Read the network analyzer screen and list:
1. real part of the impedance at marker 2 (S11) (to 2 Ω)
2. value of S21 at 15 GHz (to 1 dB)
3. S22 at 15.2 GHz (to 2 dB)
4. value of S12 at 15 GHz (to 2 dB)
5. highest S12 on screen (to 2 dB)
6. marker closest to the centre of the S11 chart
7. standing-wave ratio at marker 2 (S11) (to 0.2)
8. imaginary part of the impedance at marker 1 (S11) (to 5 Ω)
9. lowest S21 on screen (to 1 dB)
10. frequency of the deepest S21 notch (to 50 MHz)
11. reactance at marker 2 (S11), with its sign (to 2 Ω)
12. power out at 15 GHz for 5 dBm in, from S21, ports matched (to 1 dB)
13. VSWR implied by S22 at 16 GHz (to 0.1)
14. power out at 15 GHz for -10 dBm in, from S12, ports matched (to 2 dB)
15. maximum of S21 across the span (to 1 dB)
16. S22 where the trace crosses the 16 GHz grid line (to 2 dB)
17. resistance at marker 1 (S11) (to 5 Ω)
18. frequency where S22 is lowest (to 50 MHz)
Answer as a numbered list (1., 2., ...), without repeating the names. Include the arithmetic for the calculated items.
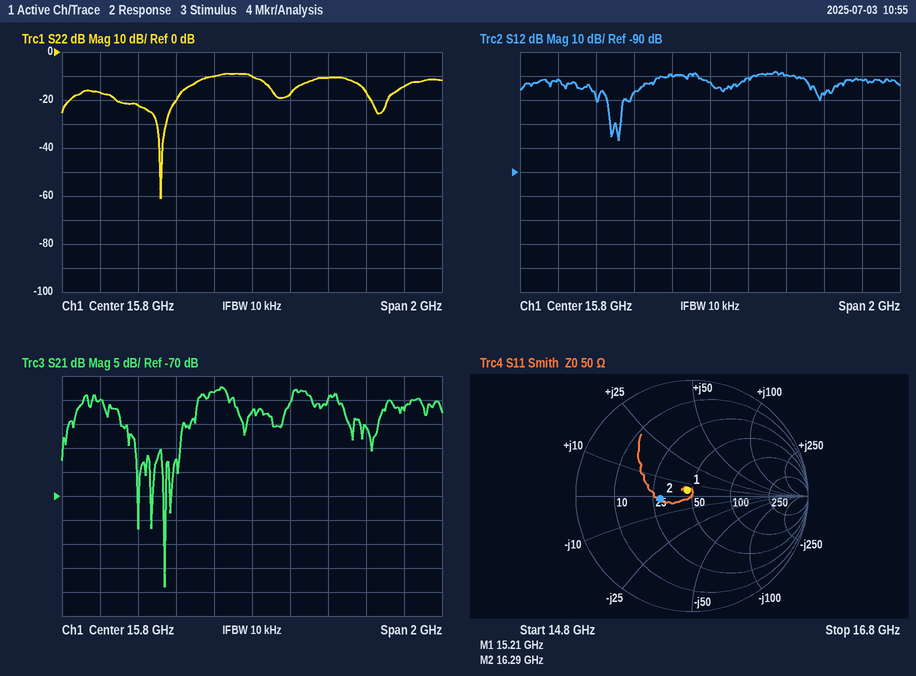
1. 28 Ω
2. -50 dB
3. -22 dB
4. -52 dB
5. -48 dB
6. marker 1
7. 1.8
8. +5 Ω
9. -89 dB
10. 15.35 GHz
11. -2 Ω
12. 5 dBm + (-50 dB) = -45 dBm
13. |Γ| = 10^(-18/20) = 0.1259; VSWR = (1 + 0.1259)/(1 − 0.1259) ≈ 1.3
14. -10 dBm + (-52 dB) = -62 dBm
15. -47 dB
16. -18 dB
17. 45 Ω
18. 15.30 GHz
